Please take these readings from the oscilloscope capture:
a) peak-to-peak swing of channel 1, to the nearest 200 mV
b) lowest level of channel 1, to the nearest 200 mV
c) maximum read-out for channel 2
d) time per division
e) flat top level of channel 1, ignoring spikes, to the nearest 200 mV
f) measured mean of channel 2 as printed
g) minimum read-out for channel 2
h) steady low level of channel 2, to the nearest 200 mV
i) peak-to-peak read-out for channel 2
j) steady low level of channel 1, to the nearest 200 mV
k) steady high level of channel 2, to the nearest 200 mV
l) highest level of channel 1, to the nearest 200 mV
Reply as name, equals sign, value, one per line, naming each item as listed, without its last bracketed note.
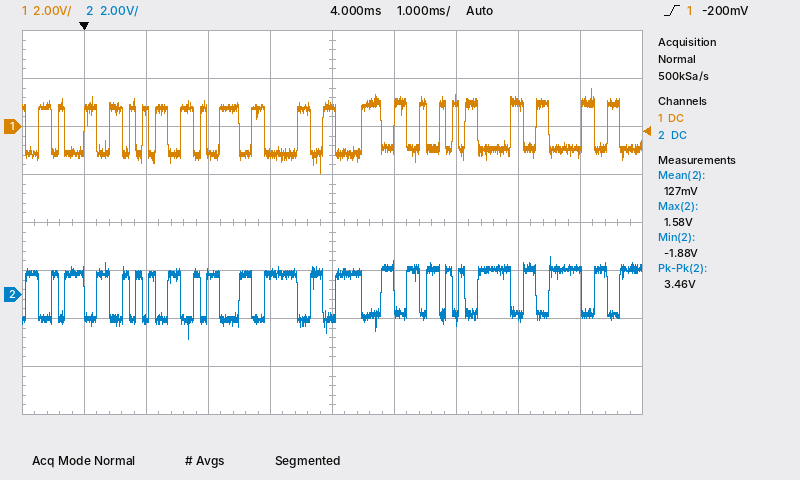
peak-to-peak swing of channel 1, to the nearest 200 mV = 3.6 V
lowest level of channel 1, to the nearest 200 mV = -2.0 V
maximum read-out for channel 2 = 1.58 V
time per division = 1 ms
flat top level of channel 1, ignoring spikes, to the nearest 200 mV = 800 mV
measured mean of channel 2 as printed = 127 mV
minimum read-out for channel 2 = -1.88 V
steady low level of channel 2, to the nearest 200 mV = -1.0 V
peak-to-peak read-out for channel 2 = 3.46 V
steady low level of channel 1, to the nearest 200 mV = -1.0 V
steady high level of channel 2, to the nearest 200 mV = 1.0 V
highest level of channel 1, to the nearest 200 mV = 1.6 V
